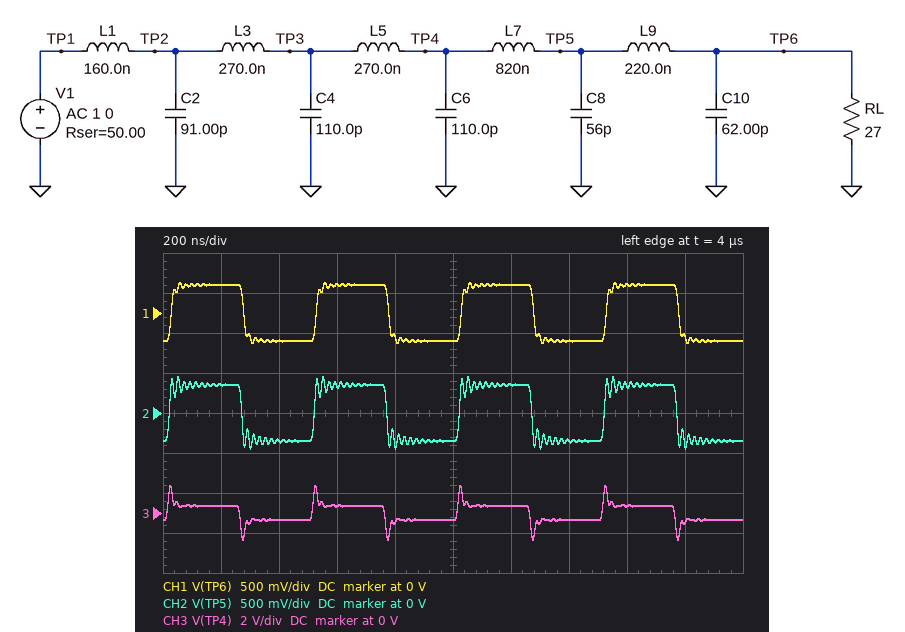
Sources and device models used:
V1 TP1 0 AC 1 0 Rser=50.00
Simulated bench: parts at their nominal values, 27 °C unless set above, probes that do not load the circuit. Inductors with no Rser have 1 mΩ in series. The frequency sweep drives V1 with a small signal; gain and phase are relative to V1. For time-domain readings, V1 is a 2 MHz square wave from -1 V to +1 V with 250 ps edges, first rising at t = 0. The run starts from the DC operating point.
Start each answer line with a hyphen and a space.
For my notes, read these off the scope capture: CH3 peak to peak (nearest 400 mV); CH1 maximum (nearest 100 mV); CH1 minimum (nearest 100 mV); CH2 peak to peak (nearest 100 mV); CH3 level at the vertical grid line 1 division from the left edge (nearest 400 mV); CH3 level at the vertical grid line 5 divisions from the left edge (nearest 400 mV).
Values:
- 2.8 V
- 400 mV
- -400 mV
- 900 mV
- 400 mV
- -400 mV
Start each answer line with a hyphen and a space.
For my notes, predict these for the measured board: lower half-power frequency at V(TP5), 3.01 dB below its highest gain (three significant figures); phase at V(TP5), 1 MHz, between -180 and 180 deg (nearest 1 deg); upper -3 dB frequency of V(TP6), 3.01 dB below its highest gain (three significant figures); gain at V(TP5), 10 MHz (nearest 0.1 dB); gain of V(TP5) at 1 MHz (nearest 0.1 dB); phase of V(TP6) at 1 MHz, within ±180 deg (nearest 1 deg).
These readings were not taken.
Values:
- 45.8 MHz
- -8 deg
- 17.0 MHz
- -9.8 dB
- -9.1 dB
- -11 deg
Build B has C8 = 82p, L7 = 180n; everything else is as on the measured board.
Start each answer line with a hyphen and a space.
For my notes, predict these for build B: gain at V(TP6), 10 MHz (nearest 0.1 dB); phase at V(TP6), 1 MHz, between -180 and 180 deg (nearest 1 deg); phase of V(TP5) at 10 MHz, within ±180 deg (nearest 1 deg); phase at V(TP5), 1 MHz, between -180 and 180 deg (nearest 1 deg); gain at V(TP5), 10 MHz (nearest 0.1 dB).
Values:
- -9.1 dB
- -8 deg
- -51 deg
- -5 deg
- -8.5 dB
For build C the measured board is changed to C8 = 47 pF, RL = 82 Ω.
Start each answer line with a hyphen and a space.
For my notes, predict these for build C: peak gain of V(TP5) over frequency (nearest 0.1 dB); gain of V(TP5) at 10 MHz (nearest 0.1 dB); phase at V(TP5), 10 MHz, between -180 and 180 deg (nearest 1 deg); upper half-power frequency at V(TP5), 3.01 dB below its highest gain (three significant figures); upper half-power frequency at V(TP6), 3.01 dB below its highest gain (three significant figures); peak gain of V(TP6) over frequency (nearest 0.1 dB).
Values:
- -4.1 dB
- -4.4 dB
- -87 deg
- 20.6 MHz
- 23.8 MHz
- -4.0 dB
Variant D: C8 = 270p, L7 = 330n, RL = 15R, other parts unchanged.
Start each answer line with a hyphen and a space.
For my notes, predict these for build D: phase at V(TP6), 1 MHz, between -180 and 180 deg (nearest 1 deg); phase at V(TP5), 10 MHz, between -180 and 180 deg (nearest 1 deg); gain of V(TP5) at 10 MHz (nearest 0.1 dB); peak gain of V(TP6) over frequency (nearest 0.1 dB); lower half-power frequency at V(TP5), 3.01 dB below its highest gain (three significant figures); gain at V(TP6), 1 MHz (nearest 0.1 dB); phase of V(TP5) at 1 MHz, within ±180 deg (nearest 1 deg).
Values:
- -10 deg
- -51 deg
- -9.9 dB
- -11.3 dB
- 16.5 MHz
- -12.7 dB
- -4 deg
